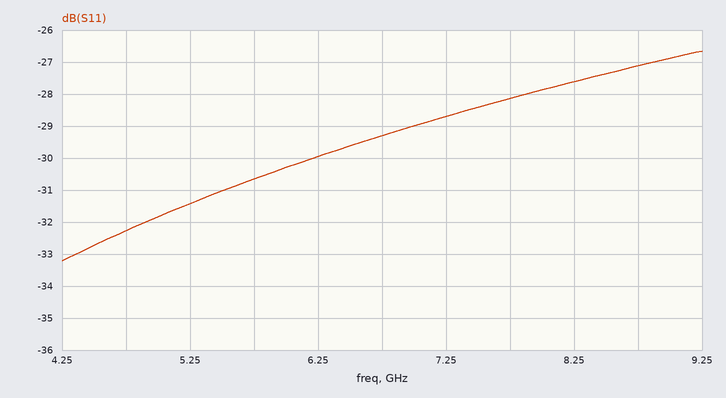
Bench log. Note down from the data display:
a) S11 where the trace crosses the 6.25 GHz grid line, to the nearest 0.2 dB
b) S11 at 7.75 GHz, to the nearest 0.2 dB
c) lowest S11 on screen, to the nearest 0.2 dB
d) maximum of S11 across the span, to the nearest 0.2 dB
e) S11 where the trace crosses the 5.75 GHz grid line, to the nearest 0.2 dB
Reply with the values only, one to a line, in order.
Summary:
-30.0 dB
-28.2 dB
-33.2 dB
-26.6 dB
-30.6 dB
